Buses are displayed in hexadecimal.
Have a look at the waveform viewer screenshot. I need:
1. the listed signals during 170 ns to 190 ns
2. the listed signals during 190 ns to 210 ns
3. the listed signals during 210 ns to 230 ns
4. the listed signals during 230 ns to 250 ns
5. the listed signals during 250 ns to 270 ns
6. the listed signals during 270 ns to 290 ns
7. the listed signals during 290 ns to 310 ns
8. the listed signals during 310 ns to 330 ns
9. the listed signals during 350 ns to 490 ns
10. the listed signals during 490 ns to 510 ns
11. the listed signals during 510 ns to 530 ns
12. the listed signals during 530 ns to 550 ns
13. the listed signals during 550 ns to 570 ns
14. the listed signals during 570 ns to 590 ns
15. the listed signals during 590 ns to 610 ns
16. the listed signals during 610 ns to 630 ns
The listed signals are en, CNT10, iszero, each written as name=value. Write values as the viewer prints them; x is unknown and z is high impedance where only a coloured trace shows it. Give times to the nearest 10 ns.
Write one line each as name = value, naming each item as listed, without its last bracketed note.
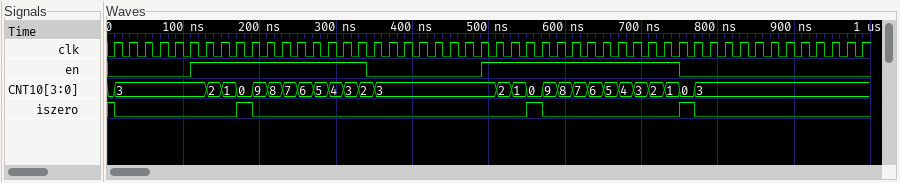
the listed signals during 170 ns to 190 ns = en=1, CNT10=0, iszero=1
the listed signals during 190 ns to 210 ns = en=1, CNT10=9, iszero=0
the listed signals during 210 ns to 230 ns = en=1, CNT10=8, iszero=0
the listed signals during 230 ns to 250 ns = en=1, CNT10=7, iszero=0
the listed signals during 250 ns to 270 ns = en=1, CNT10=6, iszero=0
the listed signals during 270 ns to 290 ns = en=1, CNT10=5, iszero=0
the listed signals during 290 ns to 310 ns = en=1, CNT10=4, iszero=0
the listed signals during 310 ns to 330 ns = en=1, CNT10=3, iszero=0
the listed signals during 350 ns to 490 ns = en=0, CNT10=3, iszero=0
the listed signals during 490 ns to 510 ns = en=1, CNT10=3, iszero=0
the listed signals during 510 ns to 530 ns = en=1, CNT10=2, iszero=0
the listed signals during 530 ns to 550 ns = en=1, CNT10=1, iszero=0
the listed signals during 550 ns to 570 ns = en=1, CNT10=0, iszero=1
the listed signals during 570 ns to 590 ns = en=1, CNT10=9, iszero=0
the listed signals during 590 ns to 610 ns = en=1, CNT10=8, iszero=0
the listed signals during 610 ns to 630 ns = en=1, CNT10=7, iszero=0
